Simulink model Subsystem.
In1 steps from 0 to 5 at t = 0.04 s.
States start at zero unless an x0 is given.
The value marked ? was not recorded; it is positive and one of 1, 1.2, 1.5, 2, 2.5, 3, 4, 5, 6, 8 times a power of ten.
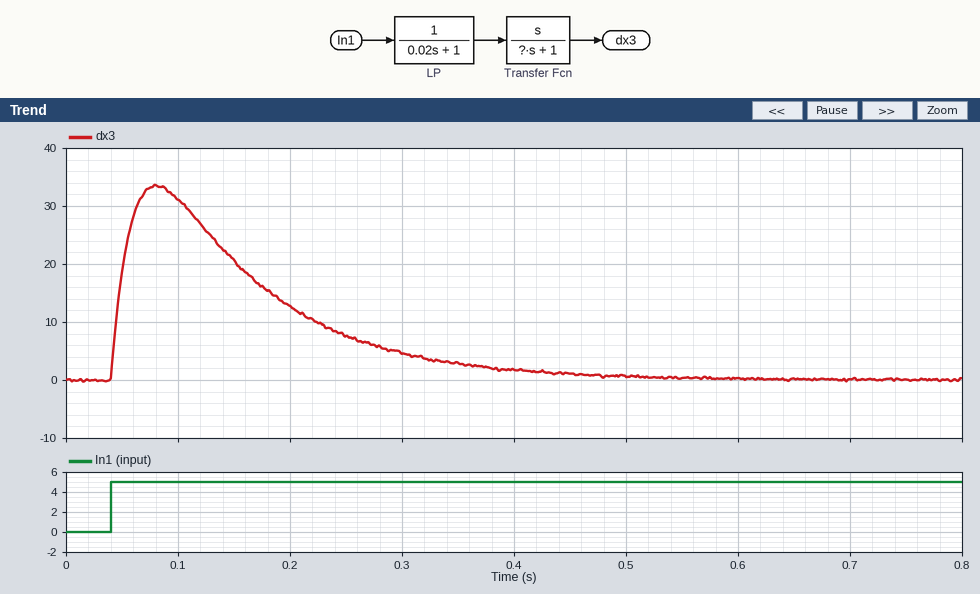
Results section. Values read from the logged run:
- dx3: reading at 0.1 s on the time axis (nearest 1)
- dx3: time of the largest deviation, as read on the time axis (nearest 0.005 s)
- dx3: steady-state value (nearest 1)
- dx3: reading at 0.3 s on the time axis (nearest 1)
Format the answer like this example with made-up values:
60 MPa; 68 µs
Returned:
31; 0.080 s; 0; 5
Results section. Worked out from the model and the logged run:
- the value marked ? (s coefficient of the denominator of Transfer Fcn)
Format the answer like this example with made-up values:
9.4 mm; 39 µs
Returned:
0.1
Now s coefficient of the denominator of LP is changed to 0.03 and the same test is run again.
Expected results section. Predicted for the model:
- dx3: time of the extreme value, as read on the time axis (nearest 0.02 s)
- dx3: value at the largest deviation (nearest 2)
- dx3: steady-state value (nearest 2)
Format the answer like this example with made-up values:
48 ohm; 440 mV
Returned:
0.10 s; 30; 0
